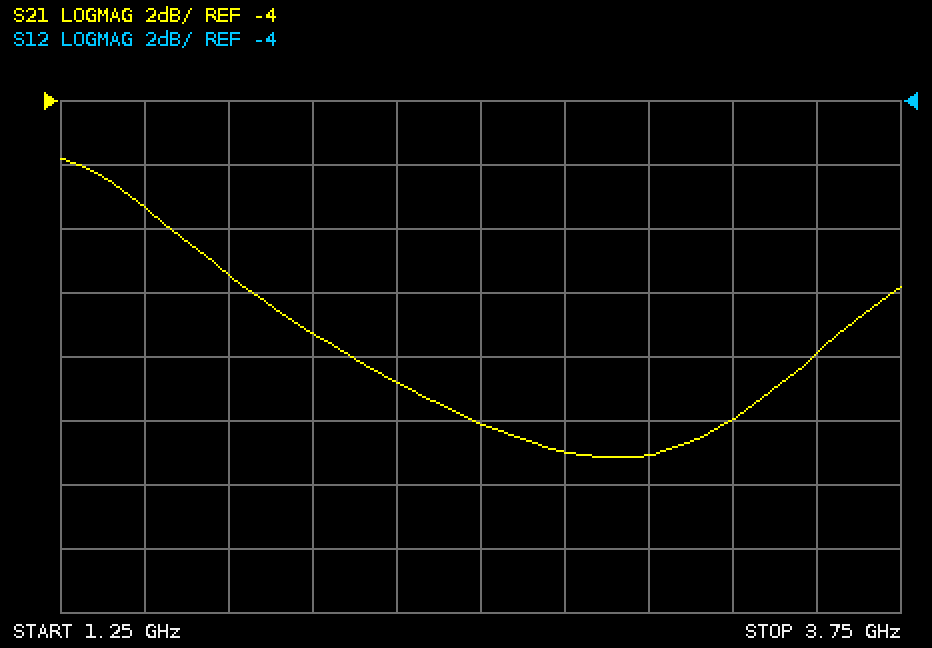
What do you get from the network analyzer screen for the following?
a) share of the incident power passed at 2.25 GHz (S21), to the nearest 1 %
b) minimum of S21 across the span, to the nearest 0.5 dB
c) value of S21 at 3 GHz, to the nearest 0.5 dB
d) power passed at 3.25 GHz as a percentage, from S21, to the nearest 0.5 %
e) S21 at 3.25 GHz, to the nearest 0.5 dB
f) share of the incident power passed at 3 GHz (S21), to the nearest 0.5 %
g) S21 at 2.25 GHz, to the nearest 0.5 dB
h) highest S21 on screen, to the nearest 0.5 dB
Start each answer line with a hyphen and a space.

- 5 %
- -15.0 dB
- -15.0 dB
- 4.0 %
- -14.0 dB
- 3.0 %
- -13.0 dB
- -6.0 dB
